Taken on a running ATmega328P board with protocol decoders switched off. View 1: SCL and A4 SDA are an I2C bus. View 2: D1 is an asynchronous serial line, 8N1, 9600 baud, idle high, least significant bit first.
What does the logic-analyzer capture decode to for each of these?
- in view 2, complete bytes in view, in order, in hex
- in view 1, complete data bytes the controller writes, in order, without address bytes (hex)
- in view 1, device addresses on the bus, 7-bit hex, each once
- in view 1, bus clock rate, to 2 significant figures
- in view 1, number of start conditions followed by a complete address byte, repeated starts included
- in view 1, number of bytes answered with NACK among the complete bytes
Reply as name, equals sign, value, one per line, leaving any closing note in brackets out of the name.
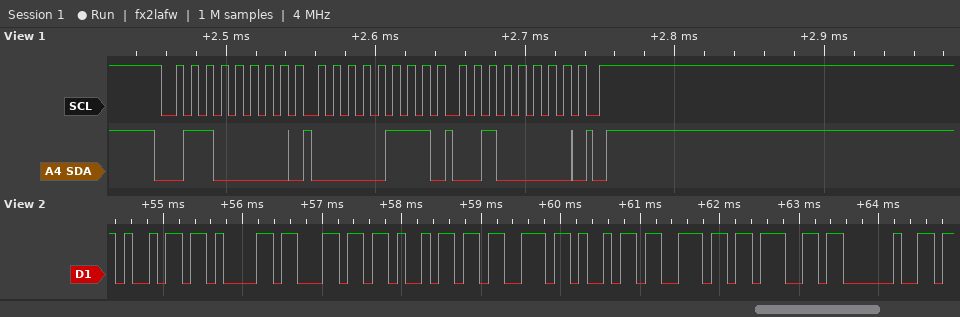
in view 2, complete bytes in view, in order, in hex = 69 61 6C 69 73 69 6E 67 20
in view 1, complete data bytes the controller writes, in order, without address bytes = 07 20
in view 1, device addresses on the bus, 7-bit hex, each once = 0x30
in view 1, bus clock rate, to 2 significant figures = 100 kHz
in view 1, number of start conditions followed by a complete address byte, repeated starts included = 1
in view 1, number of bytes answered with NACK among the complete bytes = 0
